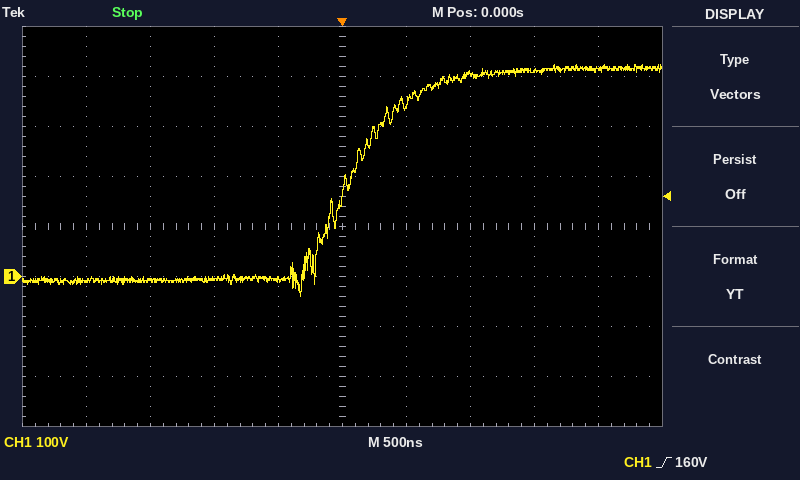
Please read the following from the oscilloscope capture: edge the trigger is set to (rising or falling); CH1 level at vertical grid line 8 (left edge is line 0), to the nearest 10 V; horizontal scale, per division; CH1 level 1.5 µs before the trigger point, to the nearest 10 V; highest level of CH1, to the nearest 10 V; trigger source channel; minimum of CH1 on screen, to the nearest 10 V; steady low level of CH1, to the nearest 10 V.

rising
410 V
500 ns
-10 V
420 V
CH1
-40 V
-10 V
